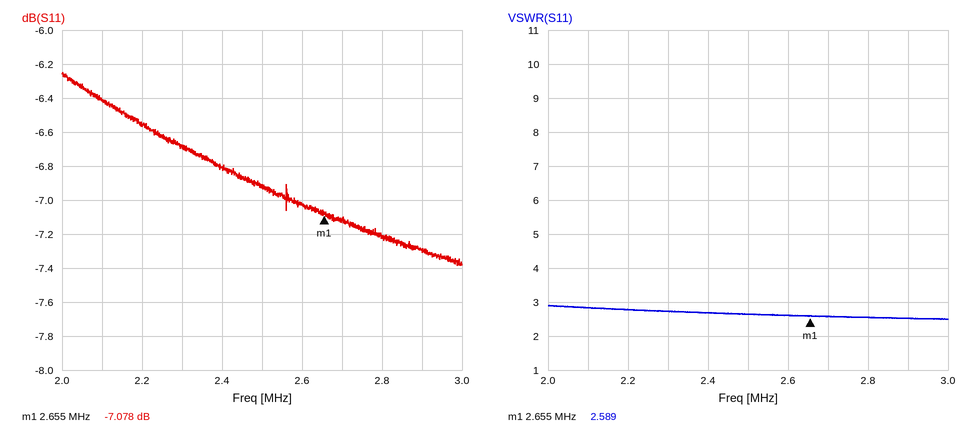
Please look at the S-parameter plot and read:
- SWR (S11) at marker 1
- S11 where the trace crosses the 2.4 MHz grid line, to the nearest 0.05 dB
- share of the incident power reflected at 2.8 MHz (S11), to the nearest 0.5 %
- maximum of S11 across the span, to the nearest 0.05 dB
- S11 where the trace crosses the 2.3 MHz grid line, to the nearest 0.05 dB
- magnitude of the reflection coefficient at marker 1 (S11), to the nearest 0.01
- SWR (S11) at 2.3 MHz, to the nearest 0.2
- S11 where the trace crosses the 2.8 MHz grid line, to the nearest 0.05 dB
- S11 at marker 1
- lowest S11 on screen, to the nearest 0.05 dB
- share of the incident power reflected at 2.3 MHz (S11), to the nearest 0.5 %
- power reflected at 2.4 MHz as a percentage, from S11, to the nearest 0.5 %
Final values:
2.589
-6.80 dB
19.0 %
-6.25 dB
-6.70 dB
0.44
2.8
-7.20 dB
-7.078 dB
-7.40 dB
21.5 %
21.0 %
